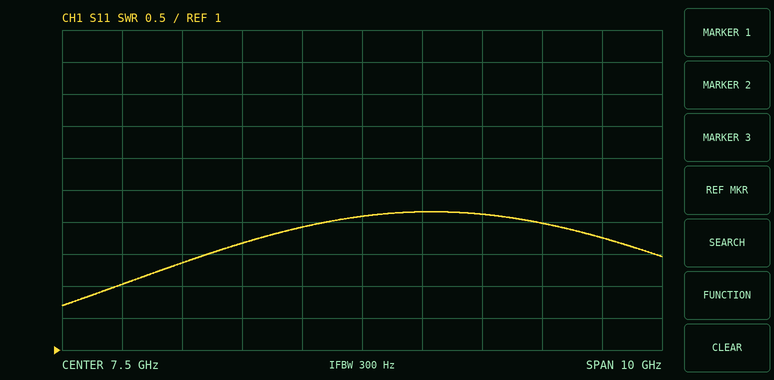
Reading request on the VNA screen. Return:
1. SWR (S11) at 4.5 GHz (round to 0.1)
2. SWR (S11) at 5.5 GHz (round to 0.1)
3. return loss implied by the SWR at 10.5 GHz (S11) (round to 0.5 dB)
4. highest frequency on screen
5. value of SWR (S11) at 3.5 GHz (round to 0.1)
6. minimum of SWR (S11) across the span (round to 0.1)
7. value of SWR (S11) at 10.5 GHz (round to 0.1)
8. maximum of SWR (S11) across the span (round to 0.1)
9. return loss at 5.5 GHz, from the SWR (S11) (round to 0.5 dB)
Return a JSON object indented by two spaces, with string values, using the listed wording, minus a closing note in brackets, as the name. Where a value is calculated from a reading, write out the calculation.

{
  "SWR (S11) at 4.5 GHz": "2.4",
  "SWR (S11) at 5.5 GHz": "2.7",
  "return loss implied by the SWR at 10.5 GHz (S11)": "−20 log10((3 − 1)/(3 + 1)) ≈ 6.0 dB",
  "highest frequency on screen": "12.5 GHz",
  "value of SWR (S11) at 3.5 GHz": "2.0",
  "minimum of SWR (S11) across the span": "1.7",
  "value of SWR (S11) at 10.5 GHz": "3.0",
  "maximum of SWR (S11) across the span": "3.2",
  "return loss at 5.5 GHz, from the SWR (S11)": "−20 log10((2.7 − 1)/(2.7 + 1)) ≈ 6.76 dB, so 7.0 dB to the nearest 0.5 dB"
}
